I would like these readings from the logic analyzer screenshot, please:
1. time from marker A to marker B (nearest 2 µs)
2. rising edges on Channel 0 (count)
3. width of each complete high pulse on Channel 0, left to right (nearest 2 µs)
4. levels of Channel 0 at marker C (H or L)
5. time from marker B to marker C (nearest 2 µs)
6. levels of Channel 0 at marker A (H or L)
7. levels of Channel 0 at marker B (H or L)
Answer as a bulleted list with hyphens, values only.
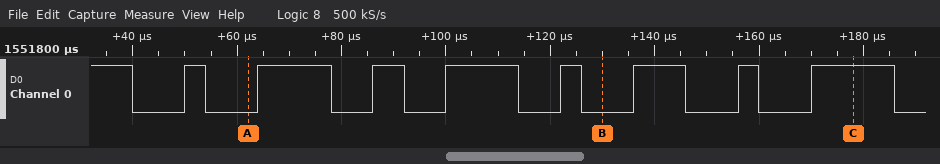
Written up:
- 68 µs
- 8
- 4 µs, 14 µs, 6 µs, 14 µs, 4 µs, 10 µs, 4 µs, 16 µs
- Channel 0=H
- 48 µs
- Channel 0=L
- Channel 0=L
